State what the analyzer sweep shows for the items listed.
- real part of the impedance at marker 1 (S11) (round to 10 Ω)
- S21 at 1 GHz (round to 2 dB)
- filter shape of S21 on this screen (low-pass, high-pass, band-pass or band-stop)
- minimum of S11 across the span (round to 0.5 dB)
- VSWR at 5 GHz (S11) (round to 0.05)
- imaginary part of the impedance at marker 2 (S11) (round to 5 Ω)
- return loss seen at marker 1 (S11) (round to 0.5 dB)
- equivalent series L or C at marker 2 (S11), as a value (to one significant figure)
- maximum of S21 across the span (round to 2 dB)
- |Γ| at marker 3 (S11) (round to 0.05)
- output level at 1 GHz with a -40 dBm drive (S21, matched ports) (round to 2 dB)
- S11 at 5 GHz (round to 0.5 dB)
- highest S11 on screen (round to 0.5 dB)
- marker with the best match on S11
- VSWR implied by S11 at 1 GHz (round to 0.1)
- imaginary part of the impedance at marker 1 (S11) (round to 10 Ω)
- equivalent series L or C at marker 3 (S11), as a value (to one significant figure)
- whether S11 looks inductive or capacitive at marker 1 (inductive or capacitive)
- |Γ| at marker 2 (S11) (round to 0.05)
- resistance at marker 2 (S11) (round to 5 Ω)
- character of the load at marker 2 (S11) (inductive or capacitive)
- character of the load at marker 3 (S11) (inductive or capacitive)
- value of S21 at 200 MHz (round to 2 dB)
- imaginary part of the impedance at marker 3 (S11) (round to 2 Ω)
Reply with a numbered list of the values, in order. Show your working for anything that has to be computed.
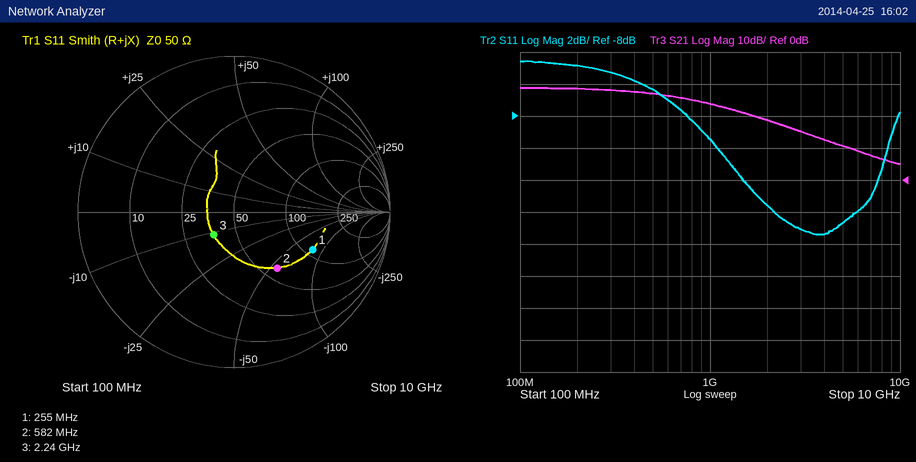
1. 110 Ω
2. 24 dB
3. low-pass
4. -15.5 dB
5. |Γ| = 10^(-14.5/20) = 0.1884; VSWR = (1 + 0.1884)/(1 − 0.1884) ≈ 1.46, so 1.45 to the nearest 0.05
6. -55 Ω
7. 5.0 dB
8. C = 1/(2π × 582 MHz × 55 Ω) ≈ 5 pF
9. 28 dB
10. 0.20
11. -40 dBm + (24 dB) = -16 dBm
12. -14.5 dB
13. -4.5 dB
14. marker 3
15. |Γ| = 10^(-9.5/20) = 0.3350; VSWR = (1 + 0.3350)/(1 − 0.3350) ≈ 2.0
16. -80 Ω
17. C = 1/(2π × 2.24 GHz × 12 Ω) ≈ 6 pF
18. capacitive
19. 0.45
20. 60 Ω
21. capacitive
22. capacitive
23. 28 dB
24. -12 Ω
